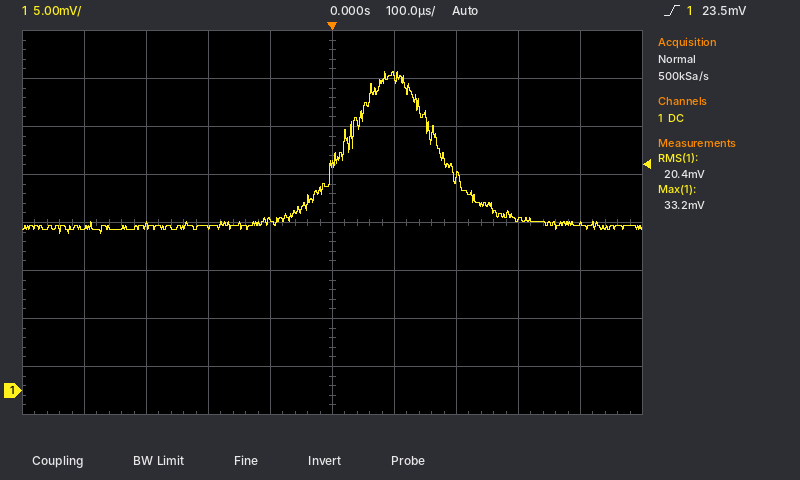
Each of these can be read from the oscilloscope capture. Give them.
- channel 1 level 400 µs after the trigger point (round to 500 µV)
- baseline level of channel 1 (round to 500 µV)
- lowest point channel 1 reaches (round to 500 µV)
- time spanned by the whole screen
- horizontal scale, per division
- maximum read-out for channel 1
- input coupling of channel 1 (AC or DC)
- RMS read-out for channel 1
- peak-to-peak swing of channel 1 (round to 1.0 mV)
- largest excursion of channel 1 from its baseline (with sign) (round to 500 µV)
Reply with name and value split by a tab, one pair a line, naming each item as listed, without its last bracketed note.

channel 1 level 400 µs after the trigger point	17.5 mV
baseline level of channel 1	17.0 mV
lowest point channel 1 reaches	16.5 mV
time spanned by the whole screen	1 ms
horizontal scale, per division	100 µs
maximum read-out for channel 1	33.2 mV
input coupling of channel 1	DC
RMS read-out for channel 1	20.4 mV
peak-to-peak swing of channel 1	17.0 mV
largest excursion of channel 1 from its baseline (with sign)	+16.0 mV
